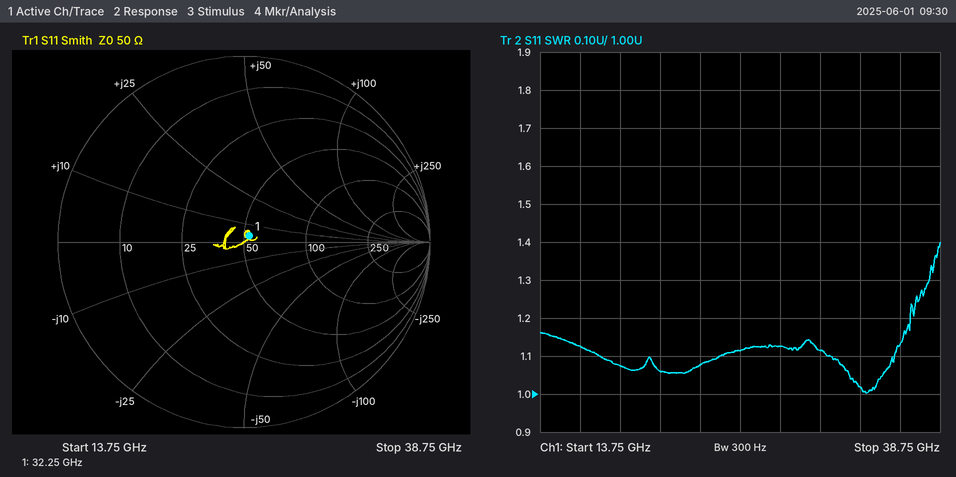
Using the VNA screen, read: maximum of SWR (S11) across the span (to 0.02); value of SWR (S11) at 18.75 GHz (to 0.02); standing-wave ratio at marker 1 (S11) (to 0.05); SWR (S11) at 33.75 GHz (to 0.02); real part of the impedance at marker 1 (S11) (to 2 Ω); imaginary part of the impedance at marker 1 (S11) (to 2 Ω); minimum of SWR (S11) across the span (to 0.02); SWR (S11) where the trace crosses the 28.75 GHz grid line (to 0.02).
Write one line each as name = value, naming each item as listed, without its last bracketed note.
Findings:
maximum of SWR (S11) across the span = 1.40
value of SWR (S11) at 18.75 GHz = 1.08
standing-wave ratio at marker 1 (S11) = 1.10
SWR (S11) at 33.75 GHz = 1.02
real part of the impedance at marker 1 (S11) = 52 Ω
imaginary part of the impedance at marker 1 (S11) = +4 Ω
minimum of SWR (S11) across the span = 1.00
SWR (S11) where the trace crosses the 28.75 GHz grid line = 1.12
